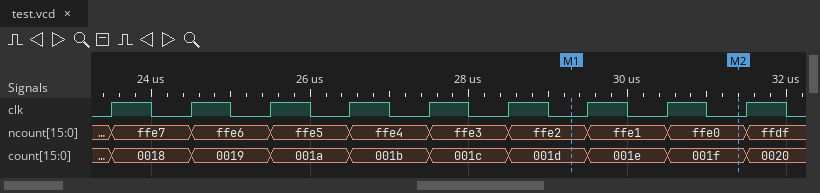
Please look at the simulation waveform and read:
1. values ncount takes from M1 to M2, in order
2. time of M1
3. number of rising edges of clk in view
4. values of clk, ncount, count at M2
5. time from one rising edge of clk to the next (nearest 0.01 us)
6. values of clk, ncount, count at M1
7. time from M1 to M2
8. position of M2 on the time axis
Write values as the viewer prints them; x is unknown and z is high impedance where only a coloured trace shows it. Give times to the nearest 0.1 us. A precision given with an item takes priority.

ffe2, ffe1, ffe0
29.3 us
9
clk=0, ncount=ffe0, count=001f
1 us
clk=0, ncount=ffe2, count=001d
2.1 us
31.4 us
